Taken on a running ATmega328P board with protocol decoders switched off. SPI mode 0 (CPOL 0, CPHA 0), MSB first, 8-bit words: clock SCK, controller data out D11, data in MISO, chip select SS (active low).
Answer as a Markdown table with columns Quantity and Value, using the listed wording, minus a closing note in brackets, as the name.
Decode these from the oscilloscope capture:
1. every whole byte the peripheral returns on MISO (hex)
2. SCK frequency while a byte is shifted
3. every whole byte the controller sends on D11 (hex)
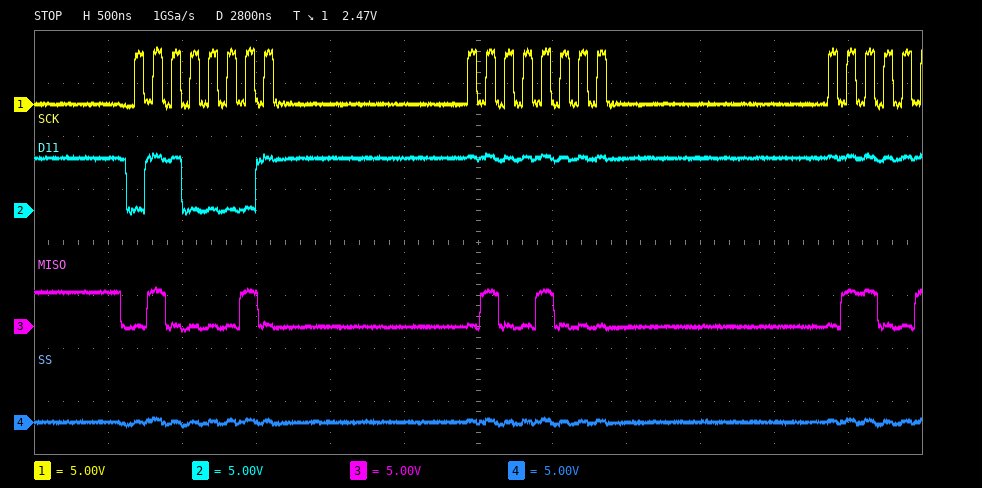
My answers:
| Quantity | Value |
|---|---|
| every whole byte the peripheral returns on MISO | 42 48 |
| SCK frequency while a byte is shifted | 8 MHz |
| every whole byte the controller sends on D11 | 61 FF |
